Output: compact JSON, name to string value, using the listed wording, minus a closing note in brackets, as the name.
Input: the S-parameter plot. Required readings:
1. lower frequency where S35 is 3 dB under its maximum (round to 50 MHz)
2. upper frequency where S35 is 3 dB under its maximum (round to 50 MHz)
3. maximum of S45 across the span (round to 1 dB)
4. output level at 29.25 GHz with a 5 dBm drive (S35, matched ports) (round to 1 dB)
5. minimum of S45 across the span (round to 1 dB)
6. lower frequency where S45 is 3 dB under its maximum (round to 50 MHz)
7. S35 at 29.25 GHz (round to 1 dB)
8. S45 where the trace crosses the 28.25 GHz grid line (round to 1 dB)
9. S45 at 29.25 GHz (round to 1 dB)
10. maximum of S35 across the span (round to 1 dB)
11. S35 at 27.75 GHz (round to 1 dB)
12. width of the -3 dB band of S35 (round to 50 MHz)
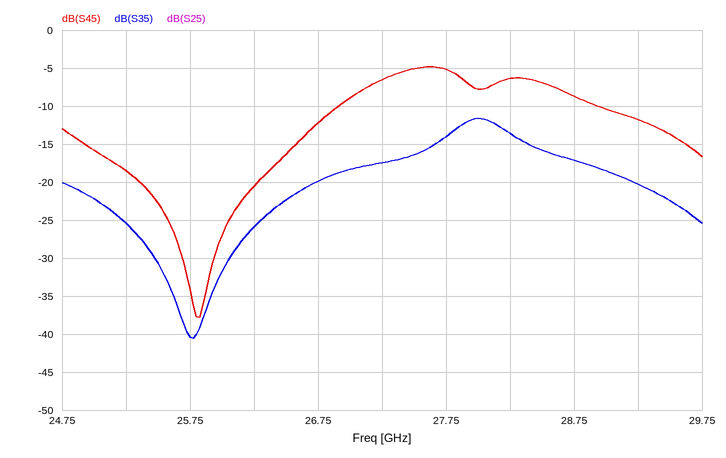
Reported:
{"lower frequency where S35 is 3 dB under its maximum": "27.70 GHz", "upper frequency where S35 is 3 dB under its maximum": "28.35 GHz", "maximum of S45 across the span": "-5 dB", "output level at 29.25 GHz with a 5 dBm drive (S35, matched ports)": "-15 dBm", "minimum of S45 across the span": "-38 dB", "lower frequency where S45 is 3 dB under its maximum": "27.10 GHz", "S35 at 29.25 GHz": "-20 dB", "S45 where the trace crosses the 28.25 GHz grid line": "-6 dB", "S45 at 29.25 GHz": "-12 dB", "maximum of S35 across the span": "-12 dB", "S35 at 27.75 GHz": "-14 dB", "width of the -3 dB band of S35": "650 MHz"}
